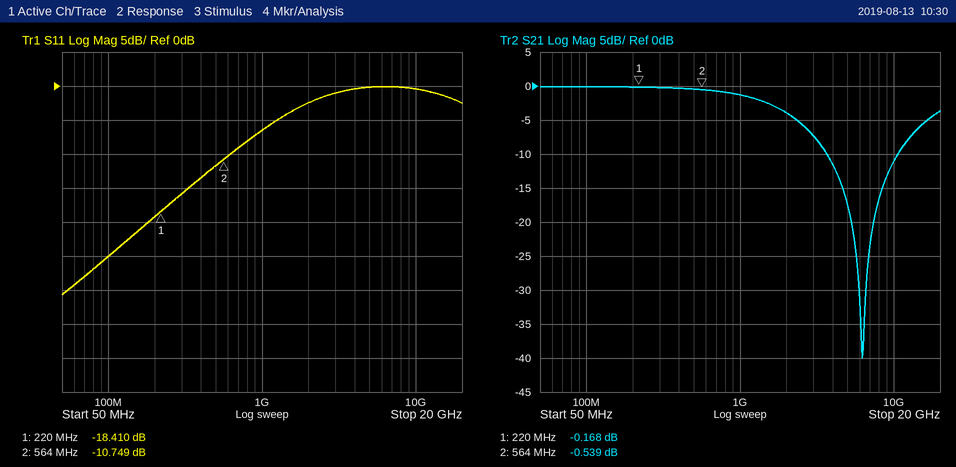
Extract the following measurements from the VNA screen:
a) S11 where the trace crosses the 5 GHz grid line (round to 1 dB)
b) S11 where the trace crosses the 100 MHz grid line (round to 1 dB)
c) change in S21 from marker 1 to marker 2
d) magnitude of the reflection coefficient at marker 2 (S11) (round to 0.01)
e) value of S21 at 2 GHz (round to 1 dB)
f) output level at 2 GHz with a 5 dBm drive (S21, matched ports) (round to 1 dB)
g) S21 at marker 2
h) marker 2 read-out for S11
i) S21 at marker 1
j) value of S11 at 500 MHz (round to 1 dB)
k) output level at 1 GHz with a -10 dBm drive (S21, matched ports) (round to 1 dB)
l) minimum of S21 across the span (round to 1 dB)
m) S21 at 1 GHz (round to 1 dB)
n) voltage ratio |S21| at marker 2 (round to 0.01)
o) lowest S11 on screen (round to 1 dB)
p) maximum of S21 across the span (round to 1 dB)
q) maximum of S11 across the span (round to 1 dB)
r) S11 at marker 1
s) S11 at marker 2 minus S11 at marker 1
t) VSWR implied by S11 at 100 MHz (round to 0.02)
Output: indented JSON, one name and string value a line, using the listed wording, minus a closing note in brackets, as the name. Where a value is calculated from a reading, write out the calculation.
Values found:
{
  "S11 where the trace crosses the 5 GHz grid line": "0 dB",
  "S11 where the trace crosses the 100 MHz grid line": "-25 dB",
  "change in S21 from marker 1 to marker 2": "-0.539 − (-0.168) = -0.371 dB",
  "magnitude of the reflection coefficient at marker 2 (S11)": "10^(-10.749/20) ≈ 0.29",
  "value of S21 at 2 GHz": "-4 dB",
  "output level at 2 GHz with a 5 dBm drive (S21, matched ports)": "5 dBm + (-4 dB) = 1 dBm",
  "S21 at marker 2": "-0.539 dB",
  "marker 2 read-out for S11": "-10.749 dB",
  "S21 at marker 1": "-0.168 dB",
  "value of S11 at 500 MHz": "-12 dB",
  "output level at 1 GHz with a -10 dBm drive (S21, matched ports)": "-10 dBm + (-1 dB) = -11 dBm",
  "minimum of S21 across the span": "-40 dB",
  "S21 at 1 GHz": "-1 dB",
  "voltage ratio |S21| at marker 2": "10^(-0.539/20) ≈ 0.94",
  "lowest S11 on screen": "-31 dB",
  "maximum of S21 across the span": "0 dB",
  "maximum of S11 across the span": "0 dB",
  "S11 at marker 1": "-18.410 dB",
  "S11 at marker 2 minus S11 at marker 1": "-10.749 − (-18.41) = 7.661 dB",
  "VSWR implied by S11 at 100 MHz": "|Γ| = 10^(-25/20) = 0.0562; VSWR = (1 + 0.0562)/(1 − 0.0562) ≈ 1.12"
}
